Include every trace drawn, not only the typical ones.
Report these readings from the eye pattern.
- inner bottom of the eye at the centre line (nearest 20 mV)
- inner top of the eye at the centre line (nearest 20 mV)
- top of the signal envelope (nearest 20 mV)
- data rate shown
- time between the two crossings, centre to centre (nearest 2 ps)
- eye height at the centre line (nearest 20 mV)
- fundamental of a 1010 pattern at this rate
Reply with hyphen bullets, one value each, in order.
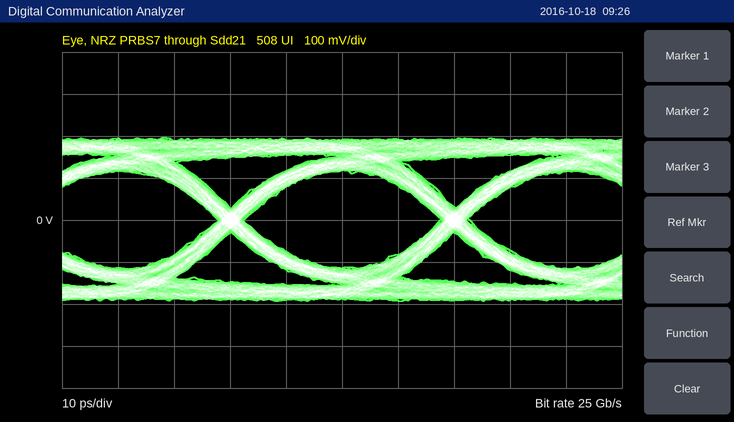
- -120 mV
- 120 mV
- 200 mV
- 25 Gb/s
- 40 ps
- 240 mV
- 12.5 GHz
